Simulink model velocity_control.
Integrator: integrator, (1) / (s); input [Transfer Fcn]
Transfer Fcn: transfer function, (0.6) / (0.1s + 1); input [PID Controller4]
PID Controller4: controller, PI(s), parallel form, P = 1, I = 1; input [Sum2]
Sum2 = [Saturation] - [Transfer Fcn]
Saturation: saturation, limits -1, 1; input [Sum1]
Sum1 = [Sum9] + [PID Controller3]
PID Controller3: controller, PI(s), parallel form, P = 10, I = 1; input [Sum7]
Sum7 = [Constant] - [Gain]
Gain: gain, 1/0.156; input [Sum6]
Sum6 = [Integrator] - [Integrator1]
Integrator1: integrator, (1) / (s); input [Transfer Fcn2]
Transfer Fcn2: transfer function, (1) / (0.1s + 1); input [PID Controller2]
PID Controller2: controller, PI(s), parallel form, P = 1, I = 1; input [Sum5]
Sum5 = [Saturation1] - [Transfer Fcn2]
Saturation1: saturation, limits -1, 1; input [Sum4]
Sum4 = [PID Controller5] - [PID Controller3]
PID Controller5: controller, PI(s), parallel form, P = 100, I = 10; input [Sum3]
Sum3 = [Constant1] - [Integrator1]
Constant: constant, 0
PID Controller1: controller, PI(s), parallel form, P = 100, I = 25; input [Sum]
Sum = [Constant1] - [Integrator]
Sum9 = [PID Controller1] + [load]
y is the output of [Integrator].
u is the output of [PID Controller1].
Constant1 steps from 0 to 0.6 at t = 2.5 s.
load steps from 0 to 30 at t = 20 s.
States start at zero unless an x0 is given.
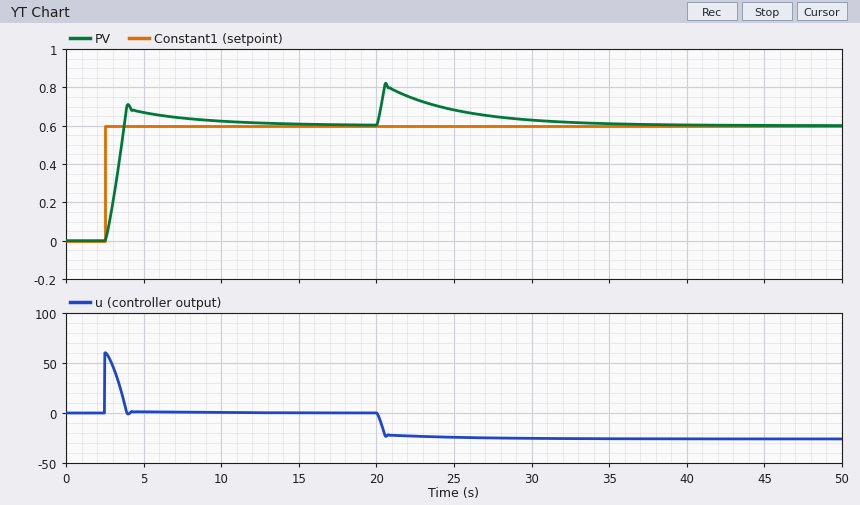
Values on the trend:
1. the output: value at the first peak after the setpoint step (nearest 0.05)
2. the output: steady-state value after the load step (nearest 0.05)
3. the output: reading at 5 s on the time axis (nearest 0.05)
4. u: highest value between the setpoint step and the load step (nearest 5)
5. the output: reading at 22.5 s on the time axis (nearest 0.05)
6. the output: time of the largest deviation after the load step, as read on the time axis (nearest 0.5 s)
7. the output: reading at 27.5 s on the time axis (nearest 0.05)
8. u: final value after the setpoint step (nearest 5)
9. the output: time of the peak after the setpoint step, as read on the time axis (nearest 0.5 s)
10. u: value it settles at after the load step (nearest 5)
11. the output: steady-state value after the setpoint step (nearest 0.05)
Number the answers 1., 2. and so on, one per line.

1. 0.70
2. 0.60
3. 0.65
4. 60
5. 0.75
6. 20.5 s
7. 0.65
8. 0
9. 4.0 s
10. -25
11. 0.60
